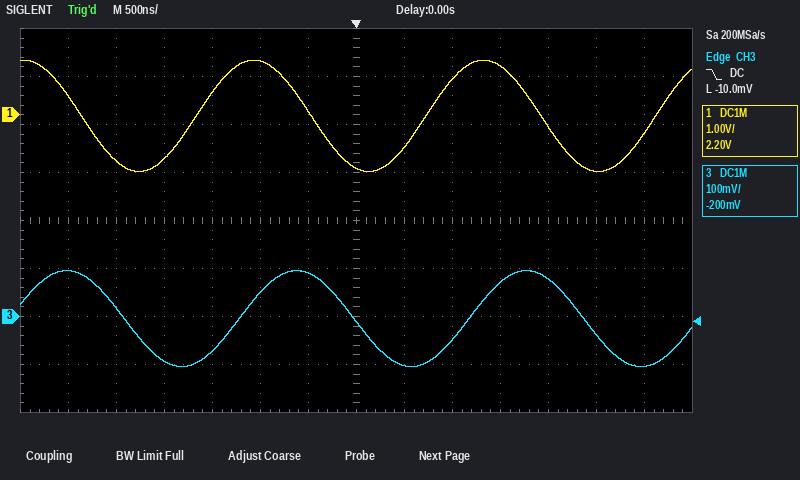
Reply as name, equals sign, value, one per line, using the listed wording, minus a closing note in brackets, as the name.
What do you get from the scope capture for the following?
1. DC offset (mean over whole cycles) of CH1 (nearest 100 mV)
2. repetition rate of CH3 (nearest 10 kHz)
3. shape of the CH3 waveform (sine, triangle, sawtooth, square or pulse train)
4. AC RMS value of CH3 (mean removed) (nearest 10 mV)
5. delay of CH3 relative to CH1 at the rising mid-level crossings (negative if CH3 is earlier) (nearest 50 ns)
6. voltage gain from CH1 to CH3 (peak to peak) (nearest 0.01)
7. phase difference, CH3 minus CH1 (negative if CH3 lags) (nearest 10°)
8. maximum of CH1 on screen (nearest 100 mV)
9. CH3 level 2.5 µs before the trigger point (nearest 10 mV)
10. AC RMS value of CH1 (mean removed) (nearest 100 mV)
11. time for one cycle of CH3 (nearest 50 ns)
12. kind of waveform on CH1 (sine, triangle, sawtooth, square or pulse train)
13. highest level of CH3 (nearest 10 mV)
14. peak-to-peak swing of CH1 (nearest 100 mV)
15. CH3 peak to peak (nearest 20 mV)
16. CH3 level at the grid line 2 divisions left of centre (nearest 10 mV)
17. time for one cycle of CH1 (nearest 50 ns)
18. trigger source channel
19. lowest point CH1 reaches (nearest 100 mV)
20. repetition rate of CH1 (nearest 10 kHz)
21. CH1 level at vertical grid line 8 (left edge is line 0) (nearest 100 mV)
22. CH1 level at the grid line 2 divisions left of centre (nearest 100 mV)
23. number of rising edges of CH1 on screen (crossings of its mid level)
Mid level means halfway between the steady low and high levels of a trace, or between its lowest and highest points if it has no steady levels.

DC offset (mean over whole cycles) of CH1 = 0.0 V
repetition rate of CH3 = 420 kHz
shape of the CH3 waveform = sine
AC RMS value of CH3 (mean removed) = 70 mV
delay of CH3 relative to CH1 at the rising mid-level crossings (negative if CH3 is earlier) = +450 ns
voltage gain from CH1 to CH3 (peak to peak) = 0.09
phase difference, CH3 minus CH1 (negative if CH3 lags) = -70°
maximum of CH1 on screen = 1.1 V
CH3 level 2.5 µs before the trigger point = 20 mV
AC RMS value of CH1 (mean removed) = 800 mV
time for one cycle of CH3 = 2.40 µs
kind of waveform on CH1 = sine
highest level of CH3 = 100 mV
peak-to-peak swing of CH1 = 2.3 V
CH3 peak to peak = 200 mV
CH3 level at the grid line 2 divisions left of centre = 50 mV
time for one cycle of CH1 = 2.40 µs
trigger source channel = CH3
lowest point CH1 reaches = -1.2 V
repetition rate of CH1 = 420 kHz
CH1 level at vertical grid line 8 (left edge is line 0) = -700 mV
CH1 level at the grid line 2 divisions left of centre = 1.1 V
number of rising edges of CH1 on screen = 3
